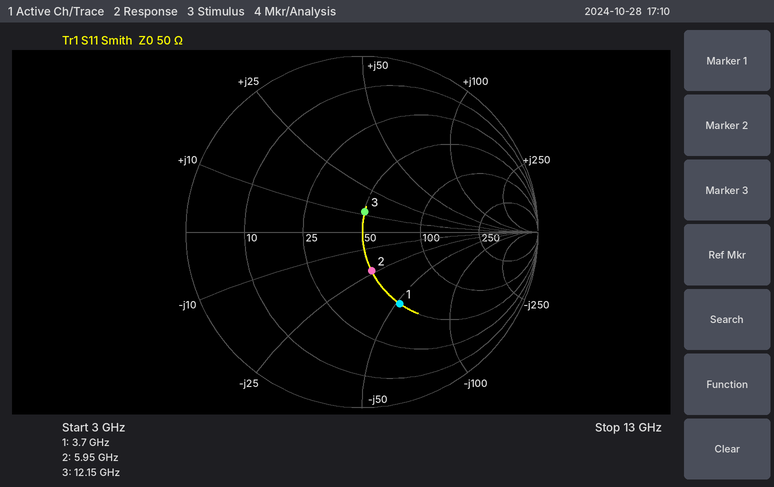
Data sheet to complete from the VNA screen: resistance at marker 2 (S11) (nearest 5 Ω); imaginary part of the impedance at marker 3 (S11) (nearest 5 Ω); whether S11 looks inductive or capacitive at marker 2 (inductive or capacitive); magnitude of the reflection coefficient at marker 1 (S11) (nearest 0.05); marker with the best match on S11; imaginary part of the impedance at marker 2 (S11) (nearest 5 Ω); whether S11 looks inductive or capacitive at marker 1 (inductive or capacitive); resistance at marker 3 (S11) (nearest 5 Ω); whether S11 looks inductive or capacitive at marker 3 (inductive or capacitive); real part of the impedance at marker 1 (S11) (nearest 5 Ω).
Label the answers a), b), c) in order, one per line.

a) 50 Ω
b) +10 Ω
c) capacitive
d) 0.45
e) marker 3
f) -25 Ω
g) capacitive
h) 50 Ω
i) inductive
j) 50 Ω
